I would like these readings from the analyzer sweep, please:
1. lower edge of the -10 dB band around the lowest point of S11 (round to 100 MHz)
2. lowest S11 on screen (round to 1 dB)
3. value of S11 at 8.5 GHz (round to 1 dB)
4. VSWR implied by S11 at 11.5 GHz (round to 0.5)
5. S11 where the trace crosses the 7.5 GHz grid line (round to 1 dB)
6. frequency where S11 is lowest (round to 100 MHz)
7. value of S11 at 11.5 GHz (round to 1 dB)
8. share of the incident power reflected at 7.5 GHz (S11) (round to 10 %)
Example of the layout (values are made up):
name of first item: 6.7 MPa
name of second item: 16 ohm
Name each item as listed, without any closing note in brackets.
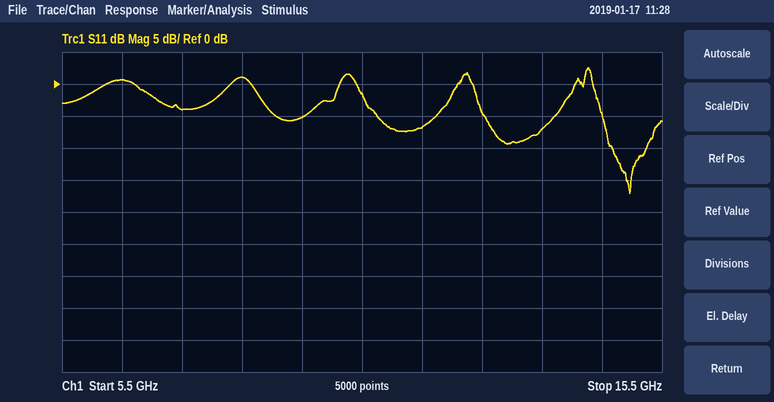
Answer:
lower edge of the -10 dB band around the lowest point of S11: 14.7 GHz
lowest S11 on screen: -17 dB
value of S11 at 8.5 GHz: 1 dB
VSWR implied by S11 at 11.5 GHz: 2.5
S11 where the trace crosses the 7.5 GHz grid line: -4 dB
frequency where S11 is lowest: 15.0 GHz
value of S11 at 11.5 GHz: -7 dB
share of the incident power reflected at 7.5 GHz (S11): 40 %
